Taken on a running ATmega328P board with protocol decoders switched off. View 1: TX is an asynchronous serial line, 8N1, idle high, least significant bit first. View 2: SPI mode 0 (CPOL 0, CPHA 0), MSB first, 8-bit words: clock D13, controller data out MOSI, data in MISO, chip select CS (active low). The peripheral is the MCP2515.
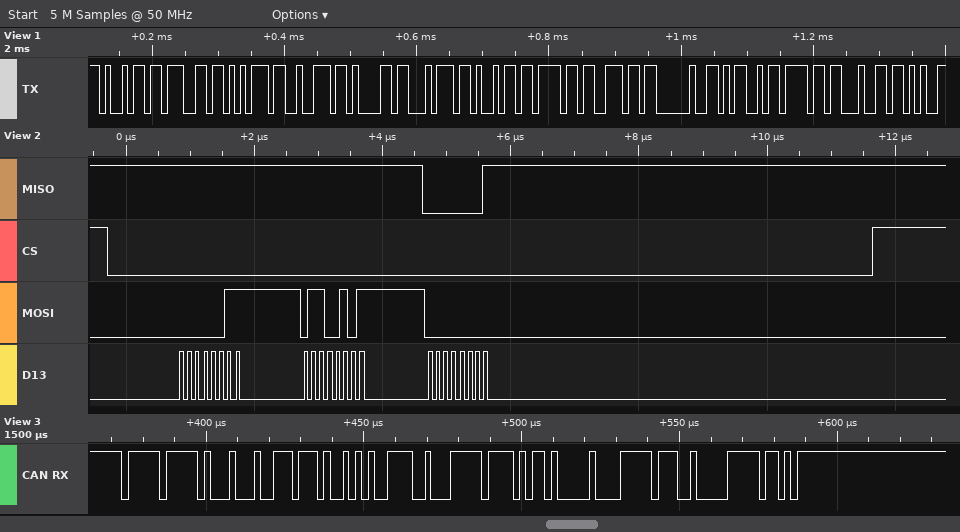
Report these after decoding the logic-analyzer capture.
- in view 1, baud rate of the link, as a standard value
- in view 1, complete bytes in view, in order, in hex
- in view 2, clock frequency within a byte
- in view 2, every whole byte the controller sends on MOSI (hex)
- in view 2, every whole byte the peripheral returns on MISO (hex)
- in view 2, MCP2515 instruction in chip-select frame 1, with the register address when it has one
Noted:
115200 baud
69 67 75 72 61 74 69 6F 6E 20 4D 6F 64
8 MHz
03 65 00
FF FF 01
READ 0x65
